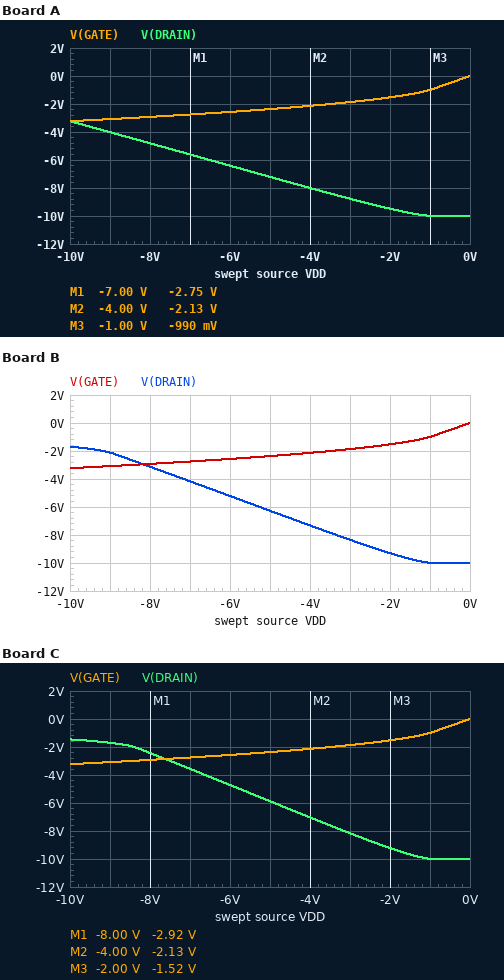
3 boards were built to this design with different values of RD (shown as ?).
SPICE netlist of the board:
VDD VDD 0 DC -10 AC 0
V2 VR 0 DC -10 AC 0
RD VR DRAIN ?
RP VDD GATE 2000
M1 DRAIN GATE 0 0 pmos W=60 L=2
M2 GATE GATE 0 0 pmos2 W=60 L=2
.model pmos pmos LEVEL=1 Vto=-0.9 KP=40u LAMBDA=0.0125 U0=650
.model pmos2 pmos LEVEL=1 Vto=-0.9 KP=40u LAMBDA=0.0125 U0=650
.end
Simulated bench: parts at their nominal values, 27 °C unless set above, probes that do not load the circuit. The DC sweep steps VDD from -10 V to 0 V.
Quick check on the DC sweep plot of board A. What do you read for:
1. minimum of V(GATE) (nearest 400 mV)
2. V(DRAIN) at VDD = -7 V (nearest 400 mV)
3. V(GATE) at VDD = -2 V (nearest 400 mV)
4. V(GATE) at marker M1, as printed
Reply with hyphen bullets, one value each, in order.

- -3.2 V
- -5.6 V
- -1.6 V
- -2.75 V
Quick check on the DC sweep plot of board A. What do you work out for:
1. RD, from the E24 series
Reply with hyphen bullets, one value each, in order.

- 2 kΩ
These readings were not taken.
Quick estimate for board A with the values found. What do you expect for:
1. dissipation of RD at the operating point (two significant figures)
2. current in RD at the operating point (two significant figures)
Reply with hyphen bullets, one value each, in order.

- 23 mW
- 3.4 mA
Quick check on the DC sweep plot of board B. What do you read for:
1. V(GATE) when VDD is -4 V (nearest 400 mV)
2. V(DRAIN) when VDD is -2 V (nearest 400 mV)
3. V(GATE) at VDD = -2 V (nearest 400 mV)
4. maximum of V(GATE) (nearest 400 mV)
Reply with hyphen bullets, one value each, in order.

- -2.0 V
- -9.2 V
- -1.6 V
- 0 V
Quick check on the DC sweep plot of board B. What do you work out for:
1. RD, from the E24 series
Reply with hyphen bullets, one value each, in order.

- 2.7 kΩ
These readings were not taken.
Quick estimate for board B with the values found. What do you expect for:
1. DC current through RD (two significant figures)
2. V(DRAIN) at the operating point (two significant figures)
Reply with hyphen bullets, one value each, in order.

- 3.1 mA
- -1.7 V
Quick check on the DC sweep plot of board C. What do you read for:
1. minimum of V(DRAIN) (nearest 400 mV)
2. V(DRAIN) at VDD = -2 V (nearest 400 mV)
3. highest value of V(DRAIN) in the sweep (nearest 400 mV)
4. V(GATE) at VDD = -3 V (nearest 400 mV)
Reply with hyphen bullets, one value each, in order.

- -10.0 V
- -9.2 V
- -1.6 V
- -2.0 V
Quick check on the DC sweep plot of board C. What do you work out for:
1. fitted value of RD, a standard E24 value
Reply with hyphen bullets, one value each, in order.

- 3 kΩ
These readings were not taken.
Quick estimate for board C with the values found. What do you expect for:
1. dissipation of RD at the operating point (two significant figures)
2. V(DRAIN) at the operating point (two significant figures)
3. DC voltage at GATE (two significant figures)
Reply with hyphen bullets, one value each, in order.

- 24 mW
- -1.5 V
- -3.2 V
